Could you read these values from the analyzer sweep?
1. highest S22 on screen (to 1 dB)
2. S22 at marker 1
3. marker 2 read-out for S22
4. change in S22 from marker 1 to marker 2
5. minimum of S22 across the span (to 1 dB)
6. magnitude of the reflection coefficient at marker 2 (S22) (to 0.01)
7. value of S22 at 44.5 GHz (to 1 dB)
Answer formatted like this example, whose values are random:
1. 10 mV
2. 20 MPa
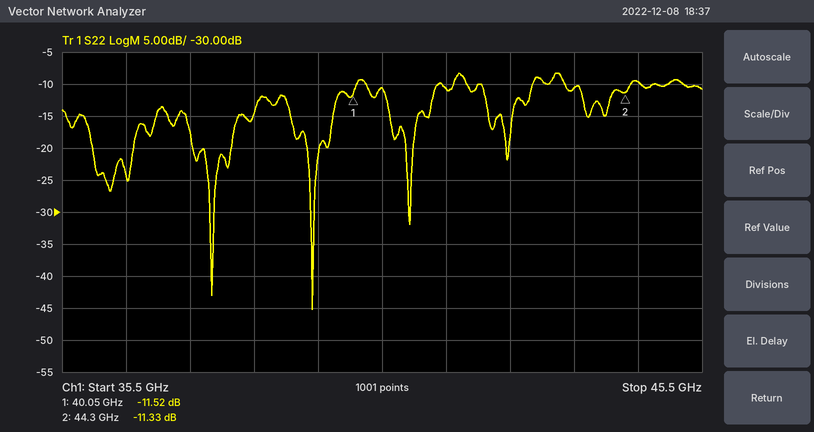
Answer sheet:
1. -8 dB
2. -11.52 dB
3. -11.33 dB
4. 0.19 dB
5. -45 dB
6. 0.27
7. -10 dB
